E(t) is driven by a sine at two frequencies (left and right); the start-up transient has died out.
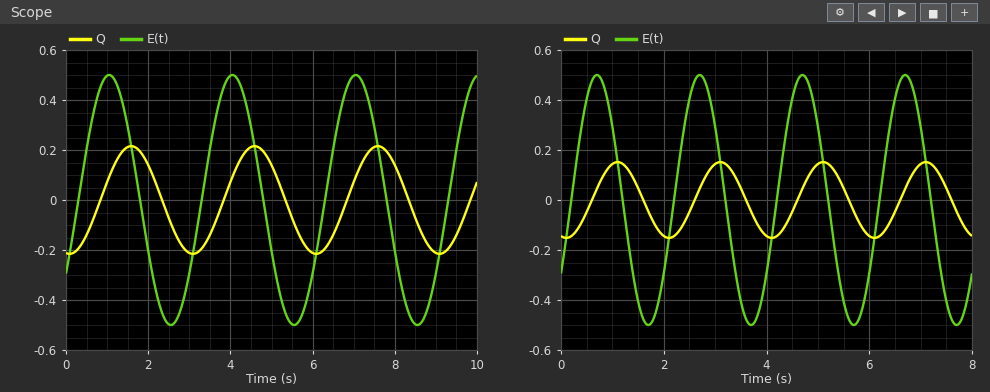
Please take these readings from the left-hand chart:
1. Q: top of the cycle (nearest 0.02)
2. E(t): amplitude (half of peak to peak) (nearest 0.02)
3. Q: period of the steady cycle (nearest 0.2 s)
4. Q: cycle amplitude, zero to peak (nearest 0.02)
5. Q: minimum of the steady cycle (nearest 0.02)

0.22
0.50
3.0 s
0.22
-0.22
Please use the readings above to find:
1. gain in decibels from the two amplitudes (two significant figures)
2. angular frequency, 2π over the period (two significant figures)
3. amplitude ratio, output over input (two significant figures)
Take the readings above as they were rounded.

-7.1 dB
2.1 rad/s
0.44
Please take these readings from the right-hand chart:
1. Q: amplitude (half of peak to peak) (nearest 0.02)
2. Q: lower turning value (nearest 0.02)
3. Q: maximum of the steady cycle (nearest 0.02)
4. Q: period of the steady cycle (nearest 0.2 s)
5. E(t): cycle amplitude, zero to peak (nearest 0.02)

0.16
-0.16
0.16
2.0 s
0.50
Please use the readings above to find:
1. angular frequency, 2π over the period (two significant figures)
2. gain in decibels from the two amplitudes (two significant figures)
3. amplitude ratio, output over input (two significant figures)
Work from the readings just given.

3.1 rad/s
-9.9 dB
0.32
